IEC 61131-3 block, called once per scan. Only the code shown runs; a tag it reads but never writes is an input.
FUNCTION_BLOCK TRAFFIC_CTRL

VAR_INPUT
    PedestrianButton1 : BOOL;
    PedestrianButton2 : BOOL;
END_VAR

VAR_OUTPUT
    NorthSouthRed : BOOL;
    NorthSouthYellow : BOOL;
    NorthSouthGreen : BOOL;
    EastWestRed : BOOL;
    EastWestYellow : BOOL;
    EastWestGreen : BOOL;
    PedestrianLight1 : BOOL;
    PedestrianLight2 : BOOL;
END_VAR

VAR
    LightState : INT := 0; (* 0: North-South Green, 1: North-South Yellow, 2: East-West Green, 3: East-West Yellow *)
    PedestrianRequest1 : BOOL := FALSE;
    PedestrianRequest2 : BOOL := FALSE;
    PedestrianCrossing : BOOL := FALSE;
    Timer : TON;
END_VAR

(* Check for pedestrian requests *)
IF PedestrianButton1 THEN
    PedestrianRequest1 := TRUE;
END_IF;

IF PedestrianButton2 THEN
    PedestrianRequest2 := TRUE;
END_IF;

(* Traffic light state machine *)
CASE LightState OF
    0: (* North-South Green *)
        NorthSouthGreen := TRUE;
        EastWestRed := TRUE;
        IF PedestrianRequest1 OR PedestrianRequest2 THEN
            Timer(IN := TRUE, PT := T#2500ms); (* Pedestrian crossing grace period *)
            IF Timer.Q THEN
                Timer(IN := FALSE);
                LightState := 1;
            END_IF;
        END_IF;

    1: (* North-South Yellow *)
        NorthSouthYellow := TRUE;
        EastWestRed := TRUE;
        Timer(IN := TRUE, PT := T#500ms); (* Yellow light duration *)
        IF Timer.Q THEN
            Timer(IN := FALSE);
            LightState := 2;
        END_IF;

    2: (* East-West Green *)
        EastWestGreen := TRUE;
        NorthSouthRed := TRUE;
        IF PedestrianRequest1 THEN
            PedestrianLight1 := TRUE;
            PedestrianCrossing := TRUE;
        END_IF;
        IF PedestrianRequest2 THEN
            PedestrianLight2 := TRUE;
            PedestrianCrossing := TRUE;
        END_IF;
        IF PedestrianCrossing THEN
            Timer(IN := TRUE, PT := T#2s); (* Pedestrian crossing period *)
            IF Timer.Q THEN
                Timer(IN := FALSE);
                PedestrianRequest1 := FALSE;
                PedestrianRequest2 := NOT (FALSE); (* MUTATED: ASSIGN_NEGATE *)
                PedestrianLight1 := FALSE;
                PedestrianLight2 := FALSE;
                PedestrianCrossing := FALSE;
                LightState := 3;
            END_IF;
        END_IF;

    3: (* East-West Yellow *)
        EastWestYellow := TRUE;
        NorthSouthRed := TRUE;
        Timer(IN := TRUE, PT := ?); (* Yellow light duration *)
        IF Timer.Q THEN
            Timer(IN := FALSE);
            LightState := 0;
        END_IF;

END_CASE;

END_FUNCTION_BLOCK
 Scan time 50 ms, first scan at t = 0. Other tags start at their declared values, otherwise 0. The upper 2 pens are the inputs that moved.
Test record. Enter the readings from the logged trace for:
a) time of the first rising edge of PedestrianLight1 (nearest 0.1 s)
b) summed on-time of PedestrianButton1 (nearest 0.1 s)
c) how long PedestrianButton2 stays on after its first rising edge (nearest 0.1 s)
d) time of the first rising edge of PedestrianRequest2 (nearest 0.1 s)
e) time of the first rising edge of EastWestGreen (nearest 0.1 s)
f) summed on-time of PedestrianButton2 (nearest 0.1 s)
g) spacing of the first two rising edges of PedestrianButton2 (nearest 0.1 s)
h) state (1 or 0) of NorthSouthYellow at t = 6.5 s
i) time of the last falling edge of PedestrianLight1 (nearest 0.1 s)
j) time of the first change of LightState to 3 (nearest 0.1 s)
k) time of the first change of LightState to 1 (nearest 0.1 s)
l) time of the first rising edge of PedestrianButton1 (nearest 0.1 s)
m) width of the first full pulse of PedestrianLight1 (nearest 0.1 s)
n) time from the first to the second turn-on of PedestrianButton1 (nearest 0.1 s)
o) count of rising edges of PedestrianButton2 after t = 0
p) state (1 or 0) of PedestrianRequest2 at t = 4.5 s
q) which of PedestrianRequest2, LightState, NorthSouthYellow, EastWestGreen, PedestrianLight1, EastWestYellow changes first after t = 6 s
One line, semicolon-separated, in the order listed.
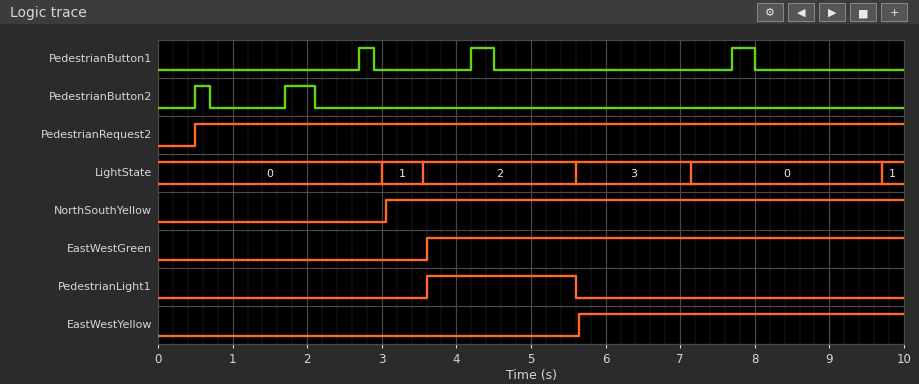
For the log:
3.6 s; 0.8 s; 0.2 s; 0.5 s; 3.6 s; 0.6 s; 1.2 s; 1; 5.6 s; 5.6 s; 3.0 s; 2.7 s; 2.0 s; 1.5 s; 2; 1; LightState
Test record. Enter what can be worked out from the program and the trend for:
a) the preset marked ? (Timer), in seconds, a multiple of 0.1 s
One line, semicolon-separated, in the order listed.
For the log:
1.5 s
